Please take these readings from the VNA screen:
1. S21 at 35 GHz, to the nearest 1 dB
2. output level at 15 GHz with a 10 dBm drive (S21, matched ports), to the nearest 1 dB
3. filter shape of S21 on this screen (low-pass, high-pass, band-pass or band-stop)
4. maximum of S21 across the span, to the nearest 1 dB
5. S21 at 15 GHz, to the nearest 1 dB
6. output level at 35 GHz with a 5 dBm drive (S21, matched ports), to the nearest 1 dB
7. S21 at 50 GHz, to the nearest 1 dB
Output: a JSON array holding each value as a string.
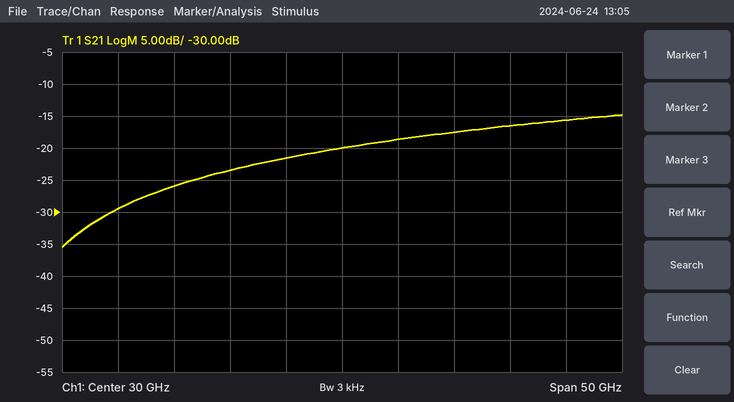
["-19 dB", "-16 dBm", "high-pass", "-15 dB", "-26 dB", "-14 dBm", "-16 dB"]
